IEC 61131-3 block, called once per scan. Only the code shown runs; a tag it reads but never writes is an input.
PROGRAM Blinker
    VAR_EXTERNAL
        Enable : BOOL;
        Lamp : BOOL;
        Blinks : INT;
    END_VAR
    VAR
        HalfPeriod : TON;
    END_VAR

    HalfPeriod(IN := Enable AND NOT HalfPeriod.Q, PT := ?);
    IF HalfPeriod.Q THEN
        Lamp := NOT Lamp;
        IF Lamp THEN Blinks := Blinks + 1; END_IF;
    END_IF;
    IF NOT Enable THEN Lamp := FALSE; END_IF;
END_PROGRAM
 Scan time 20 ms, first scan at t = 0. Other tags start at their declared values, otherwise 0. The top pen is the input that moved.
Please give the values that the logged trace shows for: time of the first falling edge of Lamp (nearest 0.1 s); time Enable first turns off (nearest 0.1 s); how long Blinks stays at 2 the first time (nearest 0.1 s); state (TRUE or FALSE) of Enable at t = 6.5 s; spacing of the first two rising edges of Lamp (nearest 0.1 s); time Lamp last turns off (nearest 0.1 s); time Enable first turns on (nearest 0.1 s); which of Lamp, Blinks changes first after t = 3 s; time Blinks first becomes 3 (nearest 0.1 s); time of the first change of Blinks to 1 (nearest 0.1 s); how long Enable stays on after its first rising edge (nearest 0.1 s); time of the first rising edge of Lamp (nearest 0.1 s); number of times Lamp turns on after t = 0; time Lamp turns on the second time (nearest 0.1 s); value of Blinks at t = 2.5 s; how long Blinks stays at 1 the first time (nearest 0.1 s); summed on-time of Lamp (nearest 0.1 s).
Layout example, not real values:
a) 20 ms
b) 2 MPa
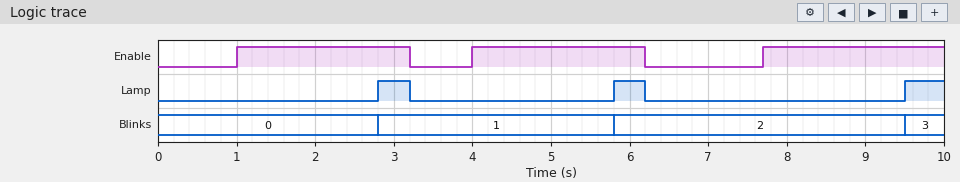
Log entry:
a) 3.2 s
b) 3.2 s
c) 3.7 s
d) FALSE
e) 3.0 s
f) 6.2 s
g) 1.0 s
h) Lamp
i) 9.5 s
j) 2.8 s
k) 2.2 s
l) 2.8 s
m) 3
n) 5.8 s
o) 0
p) 3.0 s
q) 1.3 s
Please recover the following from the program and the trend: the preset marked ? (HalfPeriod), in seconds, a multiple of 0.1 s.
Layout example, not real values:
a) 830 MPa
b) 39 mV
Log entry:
a) 1.8 s
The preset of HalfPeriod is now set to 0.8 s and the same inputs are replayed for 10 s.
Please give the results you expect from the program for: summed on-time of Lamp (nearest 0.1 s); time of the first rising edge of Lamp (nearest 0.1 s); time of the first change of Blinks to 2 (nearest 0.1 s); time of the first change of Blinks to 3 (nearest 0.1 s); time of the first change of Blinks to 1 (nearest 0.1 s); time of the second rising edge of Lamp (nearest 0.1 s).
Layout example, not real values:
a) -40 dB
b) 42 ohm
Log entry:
a) 2.5 s
b) 1.8 s
c) 4.8 s
d) 8.5 s
e) 1.8 s
f) 4.8 s
